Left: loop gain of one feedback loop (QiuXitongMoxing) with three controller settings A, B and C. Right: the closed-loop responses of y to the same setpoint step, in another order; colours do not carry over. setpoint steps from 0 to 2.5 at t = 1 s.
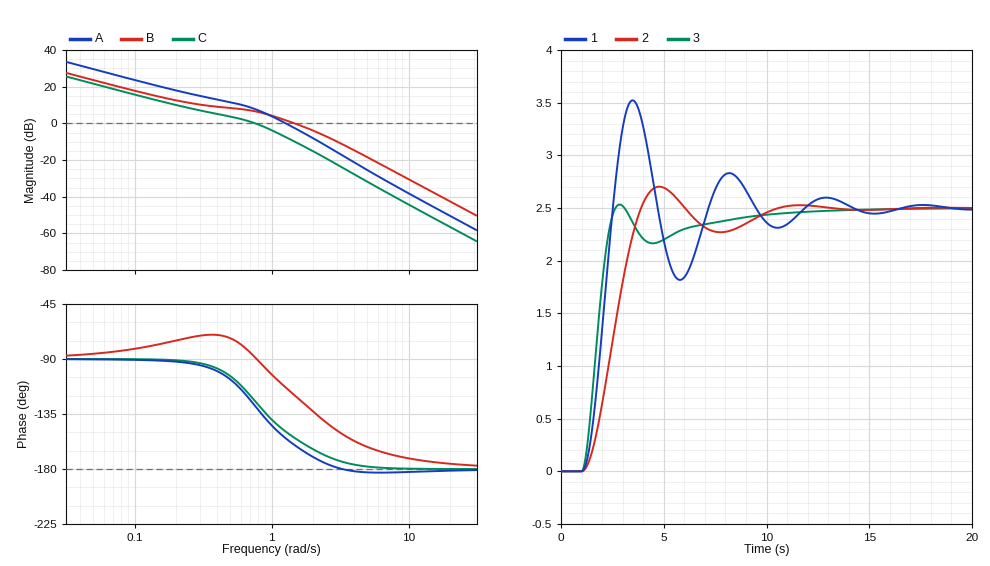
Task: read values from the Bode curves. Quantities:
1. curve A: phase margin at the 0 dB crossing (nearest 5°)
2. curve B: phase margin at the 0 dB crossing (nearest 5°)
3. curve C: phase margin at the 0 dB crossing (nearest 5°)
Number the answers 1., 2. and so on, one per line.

1. 25°
2. 60°
3. 55°
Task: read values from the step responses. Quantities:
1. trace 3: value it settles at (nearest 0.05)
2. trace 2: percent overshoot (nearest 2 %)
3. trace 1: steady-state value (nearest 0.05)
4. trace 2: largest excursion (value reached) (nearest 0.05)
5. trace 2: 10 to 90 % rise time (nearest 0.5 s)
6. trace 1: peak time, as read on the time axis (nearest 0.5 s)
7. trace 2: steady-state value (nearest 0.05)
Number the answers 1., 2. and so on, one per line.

1. 2.50
2. 8 %
3. 2.50
4. 2.70
5. 2.0 s
6. 3.5 s
7. 2.50
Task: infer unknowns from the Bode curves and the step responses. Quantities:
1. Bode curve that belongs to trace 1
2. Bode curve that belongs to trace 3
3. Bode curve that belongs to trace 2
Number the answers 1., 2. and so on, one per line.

1. A
2. B
3. C
